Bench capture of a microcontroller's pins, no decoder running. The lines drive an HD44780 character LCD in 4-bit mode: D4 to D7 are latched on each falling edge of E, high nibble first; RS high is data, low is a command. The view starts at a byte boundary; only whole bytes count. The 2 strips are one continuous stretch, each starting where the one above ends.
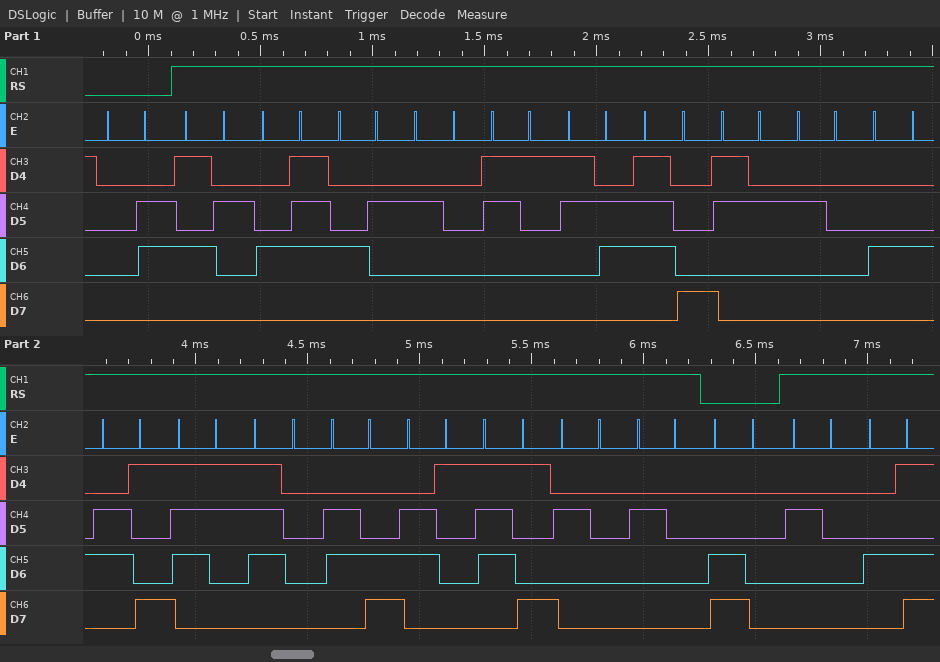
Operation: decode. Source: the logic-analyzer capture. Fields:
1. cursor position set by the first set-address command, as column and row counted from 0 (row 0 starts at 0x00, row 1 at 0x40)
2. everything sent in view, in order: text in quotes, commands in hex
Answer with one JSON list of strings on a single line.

["column 0, row 1", "0x06 \"RGB 16x2 Display  \" 0xC0 \" M\""]
